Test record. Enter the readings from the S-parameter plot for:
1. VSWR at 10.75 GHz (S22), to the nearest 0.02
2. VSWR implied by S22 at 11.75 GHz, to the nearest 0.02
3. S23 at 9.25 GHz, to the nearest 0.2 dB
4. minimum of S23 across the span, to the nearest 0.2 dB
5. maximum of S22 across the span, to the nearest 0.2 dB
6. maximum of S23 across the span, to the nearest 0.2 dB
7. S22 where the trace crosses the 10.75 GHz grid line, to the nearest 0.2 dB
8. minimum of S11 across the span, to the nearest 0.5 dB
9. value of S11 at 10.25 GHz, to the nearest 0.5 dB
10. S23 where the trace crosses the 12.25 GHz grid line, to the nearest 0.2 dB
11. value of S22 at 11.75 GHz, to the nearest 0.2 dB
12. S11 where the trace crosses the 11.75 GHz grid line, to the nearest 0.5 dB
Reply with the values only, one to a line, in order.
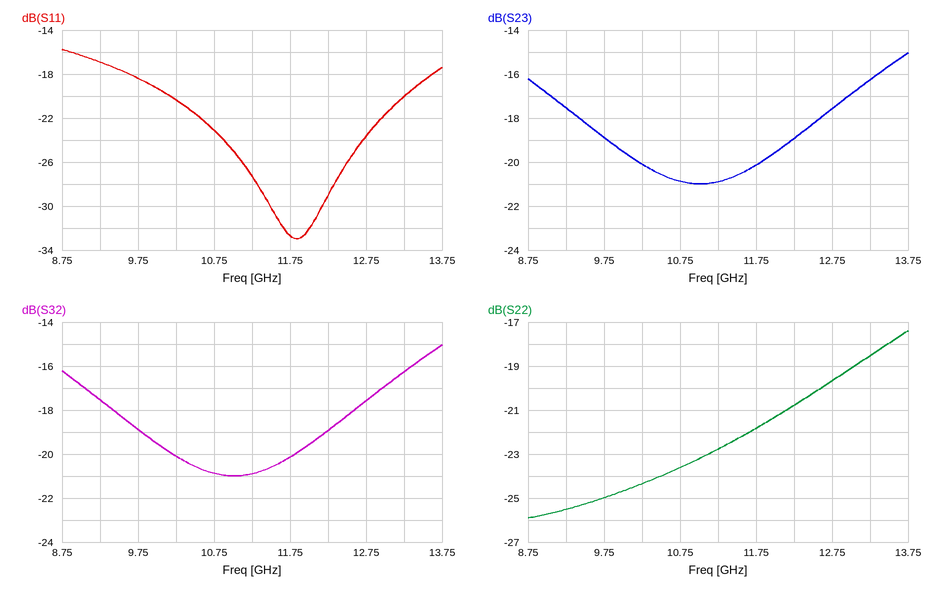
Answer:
1.14
1.18
-17.6 dB
-21.0 dB
-17.4 dB
-15.0 dB
-23.6 dB
-33.0 dB
-20.5 dB
-19.0 dB
-21.8 dB
-32.5 dB
